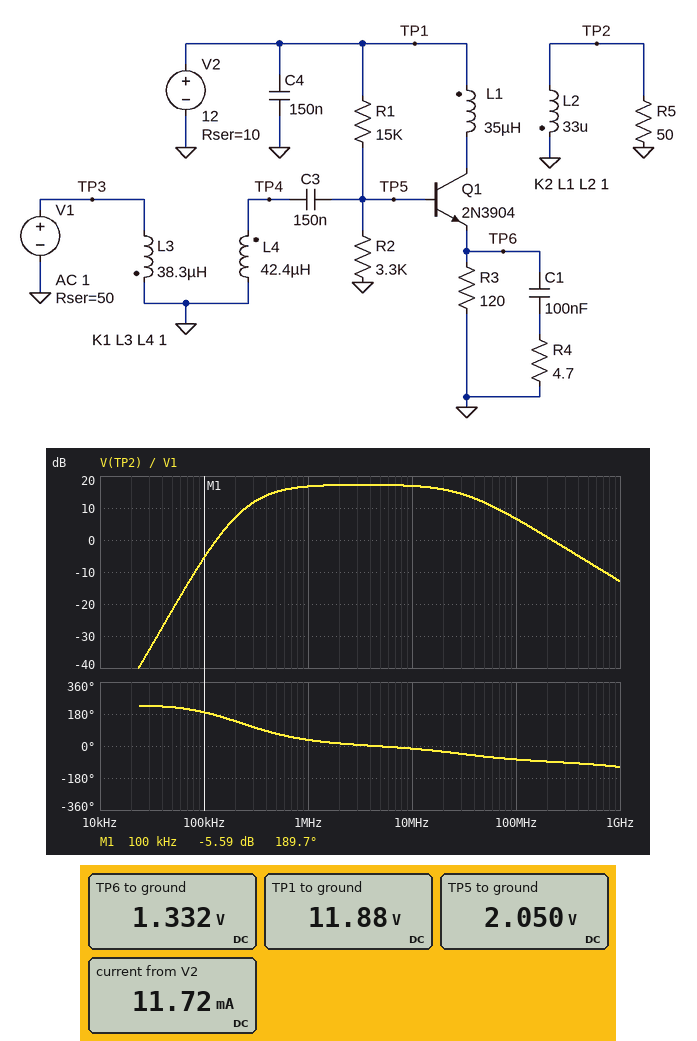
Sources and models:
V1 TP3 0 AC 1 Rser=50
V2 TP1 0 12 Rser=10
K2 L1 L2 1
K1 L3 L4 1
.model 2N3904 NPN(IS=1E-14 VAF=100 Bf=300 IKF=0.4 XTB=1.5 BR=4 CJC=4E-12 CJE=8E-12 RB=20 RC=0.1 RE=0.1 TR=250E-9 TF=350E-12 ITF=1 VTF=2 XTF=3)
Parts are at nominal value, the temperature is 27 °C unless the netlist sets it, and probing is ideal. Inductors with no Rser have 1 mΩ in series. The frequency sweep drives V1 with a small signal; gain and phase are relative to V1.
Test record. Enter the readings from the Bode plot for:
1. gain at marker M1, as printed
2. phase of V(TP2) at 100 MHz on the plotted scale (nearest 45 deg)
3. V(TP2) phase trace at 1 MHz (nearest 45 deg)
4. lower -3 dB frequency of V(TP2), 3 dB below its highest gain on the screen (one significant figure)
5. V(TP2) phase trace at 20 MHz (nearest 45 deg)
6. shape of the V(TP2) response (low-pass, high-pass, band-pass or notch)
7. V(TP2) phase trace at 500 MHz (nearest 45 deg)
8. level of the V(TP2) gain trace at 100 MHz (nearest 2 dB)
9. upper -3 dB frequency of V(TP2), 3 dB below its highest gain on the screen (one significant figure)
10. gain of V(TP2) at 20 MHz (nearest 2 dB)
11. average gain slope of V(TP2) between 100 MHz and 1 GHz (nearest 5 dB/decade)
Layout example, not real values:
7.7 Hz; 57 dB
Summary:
-5.59 dB; -90 deg; 45 deg; 400 kHz; -45 deg; band-pass; -90 deg; 6 dB; 30 MHz; 16 dB; -20 dB/decade
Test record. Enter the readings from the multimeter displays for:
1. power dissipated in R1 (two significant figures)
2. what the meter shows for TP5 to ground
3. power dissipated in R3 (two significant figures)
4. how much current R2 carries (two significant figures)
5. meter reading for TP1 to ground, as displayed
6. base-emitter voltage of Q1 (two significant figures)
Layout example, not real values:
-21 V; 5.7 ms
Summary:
6.4 mW; 2.050 V; 15 mW; 620 µA; 11.88 V; 720 mV
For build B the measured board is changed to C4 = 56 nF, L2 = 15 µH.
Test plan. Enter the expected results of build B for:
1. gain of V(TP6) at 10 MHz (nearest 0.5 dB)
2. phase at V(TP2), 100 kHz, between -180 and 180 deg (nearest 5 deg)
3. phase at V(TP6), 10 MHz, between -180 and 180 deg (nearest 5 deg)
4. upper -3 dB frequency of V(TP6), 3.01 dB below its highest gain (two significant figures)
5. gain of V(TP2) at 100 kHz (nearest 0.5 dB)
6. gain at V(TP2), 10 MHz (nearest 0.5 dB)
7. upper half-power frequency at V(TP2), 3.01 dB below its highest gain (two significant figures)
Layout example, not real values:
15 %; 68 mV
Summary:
-4.5 dB; -160 deg; 160 deg; 24 MHz; -8.5 dB; 20.0 dB; 26 MHz
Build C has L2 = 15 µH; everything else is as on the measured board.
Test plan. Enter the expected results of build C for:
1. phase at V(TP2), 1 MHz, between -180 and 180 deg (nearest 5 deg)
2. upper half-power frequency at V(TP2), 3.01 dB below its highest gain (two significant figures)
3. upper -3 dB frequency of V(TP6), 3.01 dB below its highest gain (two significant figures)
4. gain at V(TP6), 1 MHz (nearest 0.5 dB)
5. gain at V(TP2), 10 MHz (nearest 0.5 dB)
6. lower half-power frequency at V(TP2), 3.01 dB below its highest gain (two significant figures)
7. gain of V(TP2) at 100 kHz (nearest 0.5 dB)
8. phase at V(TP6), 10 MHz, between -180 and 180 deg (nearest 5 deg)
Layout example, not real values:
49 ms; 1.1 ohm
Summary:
50 deg; 26 MHz; 24 MHz; -3.5 dB; 20.0 dB; 630 kHz; -8.5 dB; 160 deg
